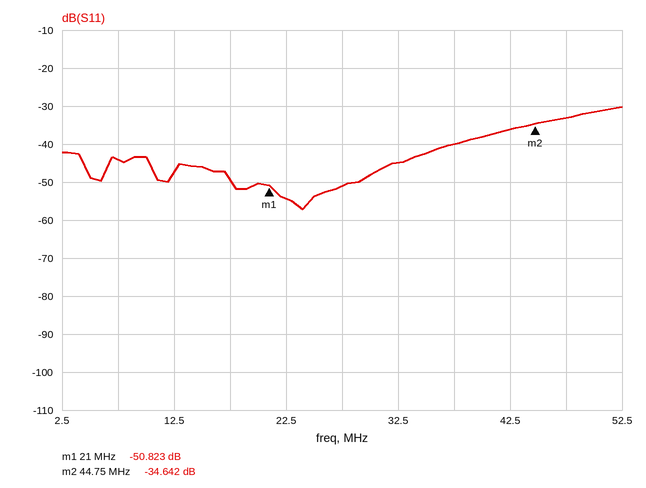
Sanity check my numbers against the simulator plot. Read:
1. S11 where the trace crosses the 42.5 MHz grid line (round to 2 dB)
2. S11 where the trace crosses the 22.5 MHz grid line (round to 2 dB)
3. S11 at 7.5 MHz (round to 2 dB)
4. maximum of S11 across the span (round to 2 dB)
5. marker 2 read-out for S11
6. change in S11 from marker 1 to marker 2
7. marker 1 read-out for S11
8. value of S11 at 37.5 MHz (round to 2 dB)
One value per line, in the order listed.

-36 dB
-54 dB
-44 dB
-30 dB
-34.642 dB
16.181 dB
-50.823 dB
-40 dB
